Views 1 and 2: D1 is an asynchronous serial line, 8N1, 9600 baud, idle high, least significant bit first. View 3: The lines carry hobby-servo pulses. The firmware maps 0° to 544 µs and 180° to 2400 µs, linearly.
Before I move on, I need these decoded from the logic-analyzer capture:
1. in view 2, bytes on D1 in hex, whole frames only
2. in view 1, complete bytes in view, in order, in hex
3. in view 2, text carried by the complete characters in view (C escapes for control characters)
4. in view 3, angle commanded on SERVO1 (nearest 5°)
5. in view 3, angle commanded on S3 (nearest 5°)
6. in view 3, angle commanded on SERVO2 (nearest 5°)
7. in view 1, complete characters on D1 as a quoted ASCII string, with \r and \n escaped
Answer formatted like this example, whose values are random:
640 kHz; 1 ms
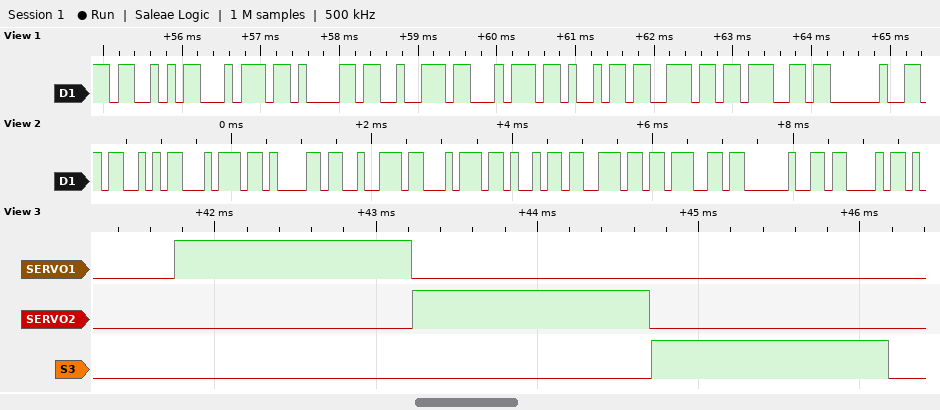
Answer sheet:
53 74 61 72 74 69 6E 67 20 43; 53 74 61 72 74 69 6E 67 20; "Starting C"; 90°; 90°; 90°; "Starting "
